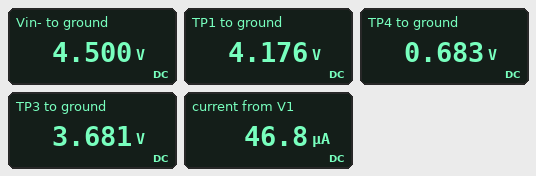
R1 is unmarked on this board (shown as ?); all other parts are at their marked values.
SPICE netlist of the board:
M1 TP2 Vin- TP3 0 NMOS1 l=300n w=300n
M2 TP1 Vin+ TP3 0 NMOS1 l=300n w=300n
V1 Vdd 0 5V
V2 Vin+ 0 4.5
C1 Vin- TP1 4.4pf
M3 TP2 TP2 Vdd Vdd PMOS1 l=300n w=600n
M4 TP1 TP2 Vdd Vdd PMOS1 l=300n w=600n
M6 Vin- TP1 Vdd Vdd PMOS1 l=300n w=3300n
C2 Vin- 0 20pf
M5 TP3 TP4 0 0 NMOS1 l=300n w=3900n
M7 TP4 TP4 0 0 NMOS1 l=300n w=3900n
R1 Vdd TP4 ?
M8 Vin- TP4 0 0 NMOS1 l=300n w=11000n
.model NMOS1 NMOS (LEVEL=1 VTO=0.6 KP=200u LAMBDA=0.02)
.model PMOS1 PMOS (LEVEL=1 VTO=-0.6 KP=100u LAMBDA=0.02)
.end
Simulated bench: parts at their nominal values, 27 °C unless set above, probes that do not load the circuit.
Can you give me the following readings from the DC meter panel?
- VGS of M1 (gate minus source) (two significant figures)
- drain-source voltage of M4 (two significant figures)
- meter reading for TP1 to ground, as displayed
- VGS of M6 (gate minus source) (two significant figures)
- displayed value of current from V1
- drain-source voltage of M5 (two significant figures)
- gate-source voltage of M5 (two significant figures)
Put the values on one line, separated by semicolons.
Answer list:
820 mV; -820 mV; 4.176 V; -820 mV; 46.8 µA; 3.7 V; 680 mV
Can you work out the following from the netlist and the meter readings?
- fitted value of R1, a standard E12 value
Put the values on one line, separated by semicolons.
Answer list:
470 kΩ
